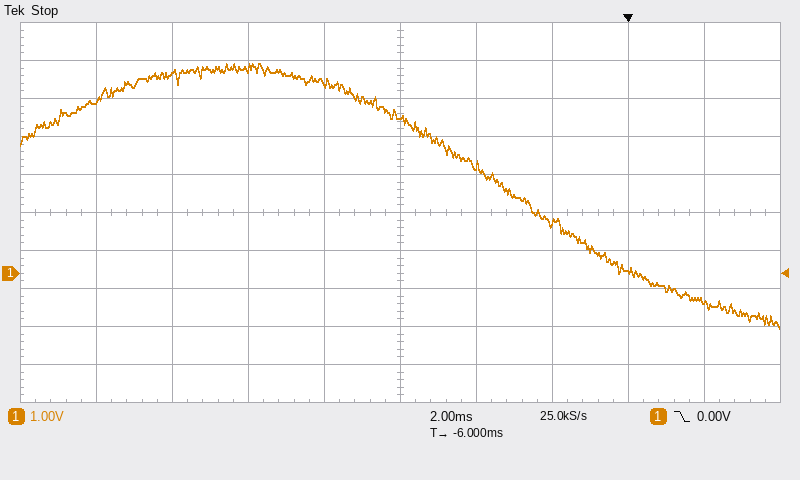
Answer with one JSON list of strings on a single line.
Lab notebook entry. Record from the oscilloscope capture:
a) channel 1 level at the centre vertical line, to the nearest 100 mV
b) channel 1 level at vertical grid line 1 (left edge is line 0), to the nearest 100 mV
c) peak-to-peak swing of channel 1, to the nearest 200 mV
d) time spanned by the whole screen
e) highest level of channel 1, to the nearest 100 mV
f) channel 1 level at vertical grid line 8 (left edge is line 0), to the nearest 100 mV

["4.1 V", "4.6 V", "7.0 V", "20 ms", "5.5 V", "100 mV"]
